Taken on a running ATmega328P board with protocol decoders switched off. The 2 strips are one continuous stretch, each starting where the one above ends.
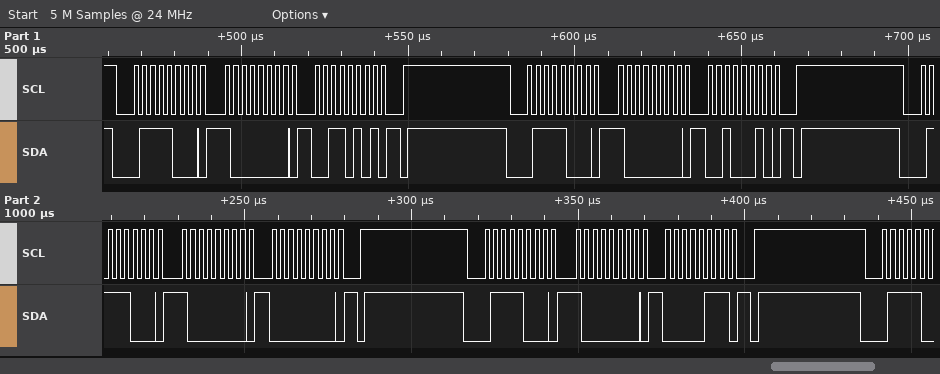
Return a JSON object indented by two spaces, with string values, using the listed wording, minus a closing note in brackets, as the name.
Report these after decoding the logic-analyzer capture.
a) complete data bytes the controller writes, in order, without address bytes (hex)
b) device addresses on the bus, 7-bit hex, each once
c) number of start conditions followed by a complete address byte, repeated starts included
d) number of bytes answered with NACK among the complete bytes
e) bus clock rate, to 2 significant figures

{
  "complete data bytes the controller writes, in order, without address bytes": "80 35 80 22 80 00 80 07",
  "device addresses on the bus, 7-bit hex, each once": "0x3C",
  "number of start conditions followed by a complete address byte, repeated starts included": "4",
  "number of bytes answered with NACK among the complete bytes": "0",
  "bus clock rate, to 2 significant figures": "400 kHz"
}
